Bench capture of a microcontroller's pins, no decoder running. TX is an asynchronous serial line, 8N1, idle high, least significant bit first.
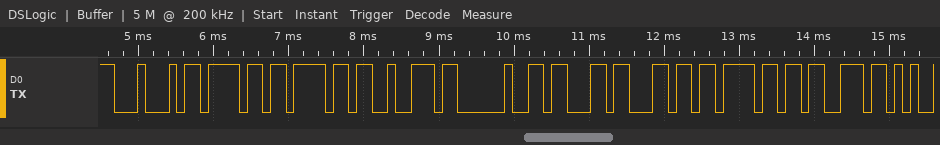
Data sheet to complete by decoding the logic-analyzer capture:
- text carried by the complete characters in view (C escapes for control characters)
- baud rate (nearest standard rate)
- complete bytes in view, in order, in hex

"Door clos"
9600 baud
0x44 0x6F 0x6F 0x72 0x20 0x63 0x6C 0x6F 0x73
